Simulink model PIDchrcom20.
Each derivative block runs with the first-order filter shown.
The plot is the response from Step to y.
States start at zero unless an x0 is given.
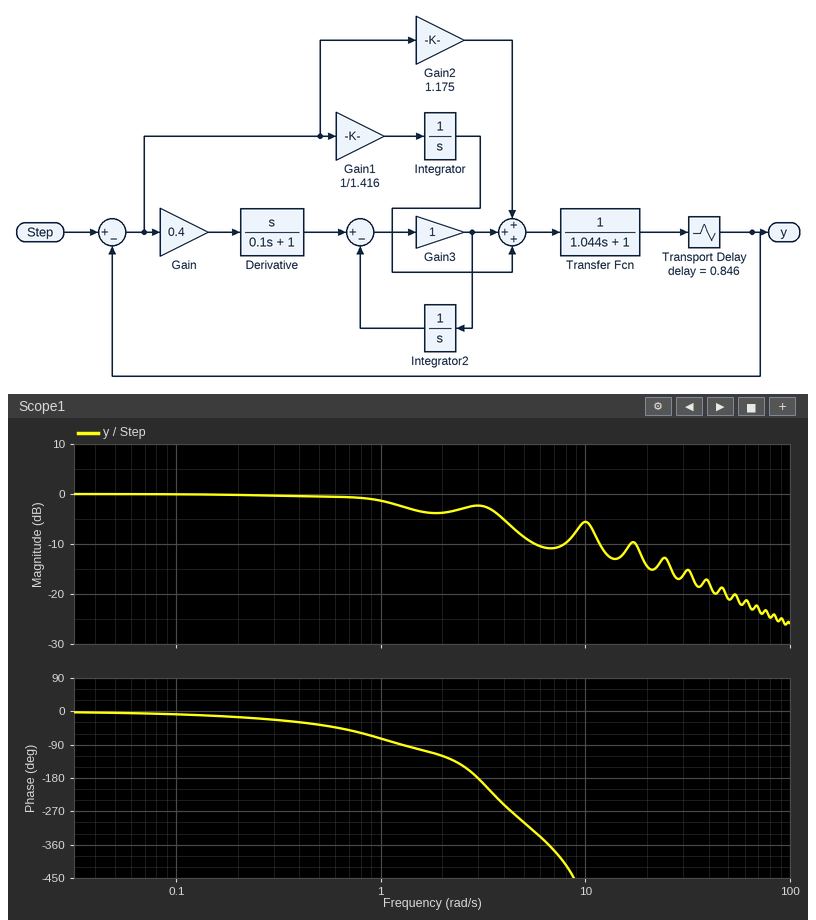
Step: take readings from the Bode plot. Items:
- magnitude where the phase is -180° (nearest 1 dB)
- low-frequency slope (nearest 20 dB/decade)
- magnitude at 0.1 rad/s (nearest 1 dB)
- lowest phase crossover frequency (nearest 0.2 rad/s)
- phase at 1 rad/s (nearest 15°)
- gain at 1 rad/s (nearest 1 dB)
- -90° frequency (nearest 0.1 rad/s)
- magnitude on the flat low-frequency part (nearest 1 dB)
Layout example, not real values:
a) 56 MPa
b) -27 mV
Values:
a) -2 dB
b) 0 dB/decade
c) 0 dB
d) 3.0 rad/s
e) -75°
f) -1 dB
g) 1.3 rad/s
h) 0 dB
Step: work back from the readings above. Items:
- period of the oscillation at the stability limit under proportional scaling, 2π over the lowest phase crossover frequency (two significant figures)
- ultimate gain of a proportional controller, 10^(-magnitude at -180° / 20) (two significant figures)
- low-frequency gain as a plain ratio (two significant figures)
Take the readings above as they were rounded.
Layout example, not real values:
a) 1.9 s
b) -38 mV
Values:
a) 2.1 s
b) 1.3
c) 1.0
